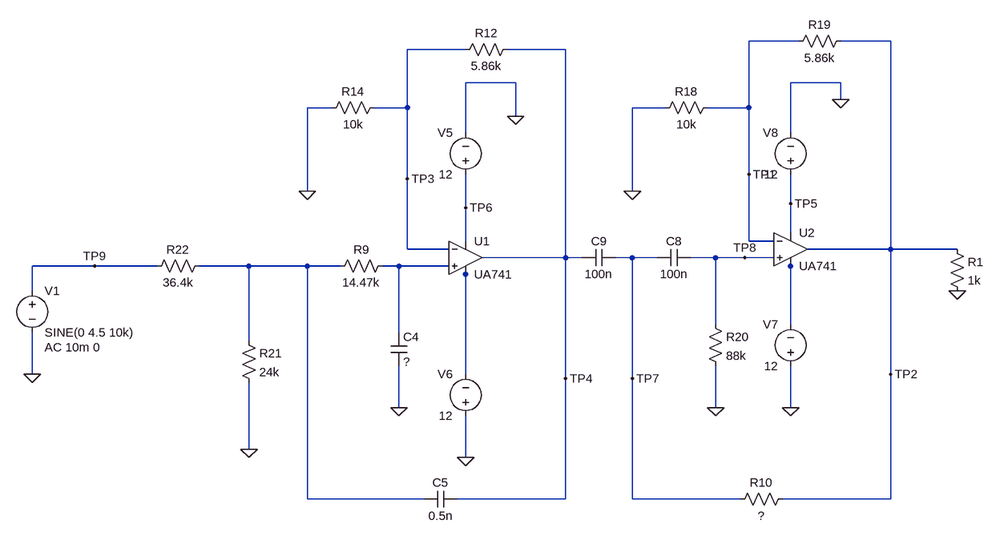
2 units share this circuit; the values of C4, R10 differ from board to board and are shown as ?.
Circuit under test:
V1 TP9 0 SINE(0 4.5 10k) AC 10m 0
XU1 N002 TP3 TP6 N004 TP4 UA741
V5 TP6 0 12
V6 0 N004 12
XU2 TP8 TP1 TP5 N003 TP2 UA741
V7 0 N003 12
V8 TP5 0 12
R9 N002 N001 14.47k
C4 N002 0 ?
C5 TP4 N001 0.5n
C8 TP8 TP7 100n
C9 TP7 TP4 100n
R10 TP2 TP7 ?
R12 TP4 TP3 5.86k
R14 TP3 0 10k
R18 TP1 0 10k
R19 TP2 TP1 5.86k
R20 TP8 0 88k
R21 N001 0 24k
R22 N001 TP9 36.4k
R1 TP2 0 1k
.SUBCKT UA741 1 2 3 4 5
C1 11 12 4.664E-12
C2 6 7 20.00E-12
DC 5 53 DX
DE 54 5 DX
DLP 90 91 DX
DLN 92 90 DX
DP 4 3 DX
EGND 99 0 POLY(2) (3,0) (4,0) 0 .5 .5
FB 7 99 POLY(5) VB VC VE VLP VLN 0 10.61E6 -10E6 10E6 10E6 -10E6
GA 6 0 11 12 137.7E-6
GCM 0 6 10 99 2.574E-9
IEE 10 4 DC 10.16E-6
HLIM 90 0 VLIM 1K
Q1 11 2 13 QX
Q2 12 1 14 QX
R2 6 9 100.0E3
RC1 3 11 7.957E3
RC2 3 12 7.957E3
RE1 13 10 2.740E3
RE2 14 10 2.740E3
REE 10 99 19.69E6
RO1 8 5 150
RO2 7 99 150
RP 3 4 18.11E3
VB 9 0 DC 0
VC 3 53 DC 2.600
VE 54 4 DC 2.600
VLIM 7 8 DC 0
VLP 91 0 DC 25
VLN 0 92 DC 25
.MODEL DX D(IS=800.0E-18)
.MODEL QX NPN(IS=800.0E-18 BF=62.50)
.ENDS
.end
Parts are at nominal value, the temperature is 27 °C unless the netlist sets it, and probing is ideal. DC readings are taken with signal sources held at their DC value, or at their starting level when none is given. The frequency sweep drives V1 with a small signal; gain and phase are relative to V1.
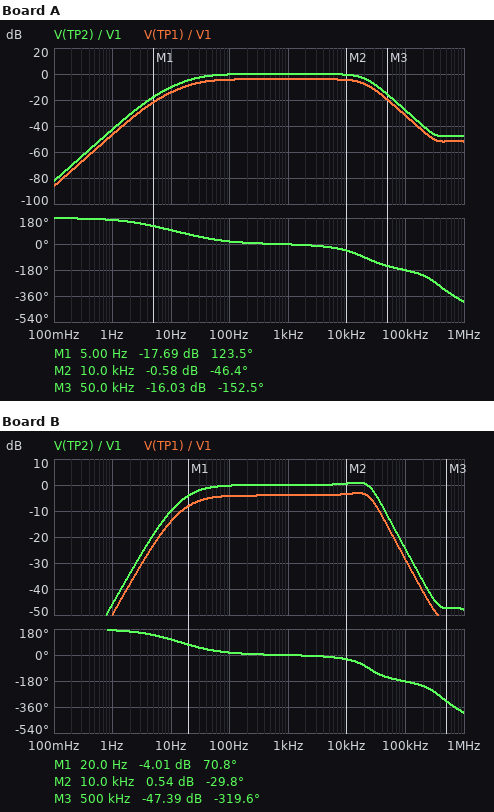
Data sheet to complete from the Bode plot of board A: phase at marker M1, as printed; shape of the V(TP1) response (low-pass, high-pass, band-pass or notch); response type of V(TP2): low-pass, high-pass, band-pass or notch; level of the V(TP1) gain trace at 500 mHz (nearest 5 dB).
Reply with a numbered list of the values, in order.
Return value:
1. 123.5 deg
2. band-pass
3. band-pass
4. -60 dB
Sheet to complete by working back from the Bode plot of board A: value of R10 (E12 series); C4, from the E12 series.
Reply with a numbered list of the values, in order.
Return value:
1. 220 kΩ
2. 560 pF
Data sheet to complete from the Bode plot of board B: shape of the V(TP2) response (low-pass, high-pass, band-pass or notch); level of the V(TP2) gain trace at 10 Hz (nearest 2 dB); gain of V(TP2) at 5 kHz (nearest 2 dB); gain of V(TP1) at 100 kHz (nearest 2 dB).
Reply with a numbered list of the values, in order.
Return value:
1. band-pass
2. -10 dB
3. 0 dB
4. -28 dB
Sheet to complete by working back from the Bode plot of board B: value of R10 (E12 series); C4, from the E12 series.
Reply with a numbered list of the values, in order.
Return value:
1. 150 kΩ
2. 390 pF
